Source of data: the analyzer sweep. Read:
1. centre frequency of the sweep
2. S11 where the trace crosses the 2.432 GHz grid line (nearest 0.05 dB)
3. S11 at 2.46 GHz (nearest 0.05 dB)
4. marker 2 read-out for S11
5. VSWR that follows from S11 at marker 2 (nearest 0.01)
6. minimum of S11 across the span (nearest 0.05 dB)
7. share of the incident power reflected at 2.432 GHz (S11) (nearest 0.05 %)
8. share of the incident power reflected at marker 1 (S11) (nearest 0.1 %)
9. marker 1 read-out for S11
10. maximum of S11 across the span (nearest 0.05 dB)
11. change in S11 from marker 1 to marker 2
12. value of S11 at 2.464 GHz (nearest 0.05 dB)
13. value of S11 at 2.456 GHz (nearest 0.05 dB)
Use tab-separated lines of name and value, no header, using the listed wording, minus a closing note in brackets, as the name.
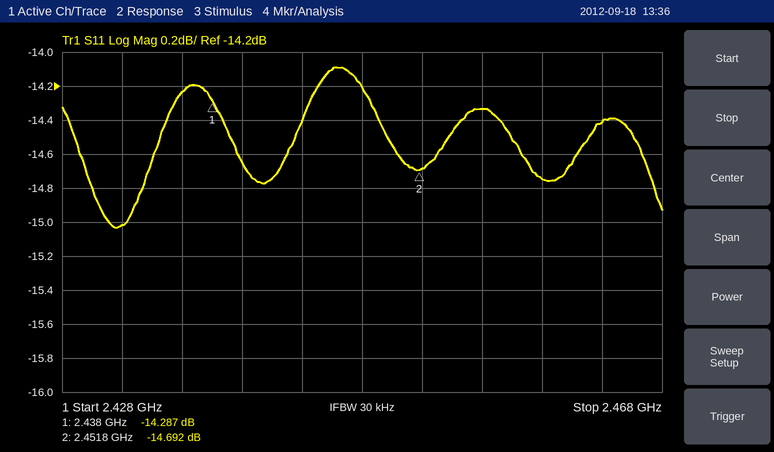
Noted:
centre frequency of the sweep	2.448 GHz
S11 where the trace crosses the 2.432 GHz grid line	-15.00 dB
S11 at 2.46 GHz	-14.75 dB
marker 2 read-out for S11	-14.692 dB
VSWR that follows from S11 at marker 2	1.45
minimum of S11 across the span	-15.05 dB
share of the incident power reflected at 2.432 GHz (S11)	3.15 %
share of the incident power reflected at marker 1 (S11)	3.7 %
marker 1 read-out for S11	-14.287 dB
maximum of S11 across the span	-14.10 dB
change in S11 from marker 1 to marker 2	-0.405 dB
value of S11 at 2.464 GHz	-14.40 dB
value of S11 at 2.456 GHz	-14.35 dB
